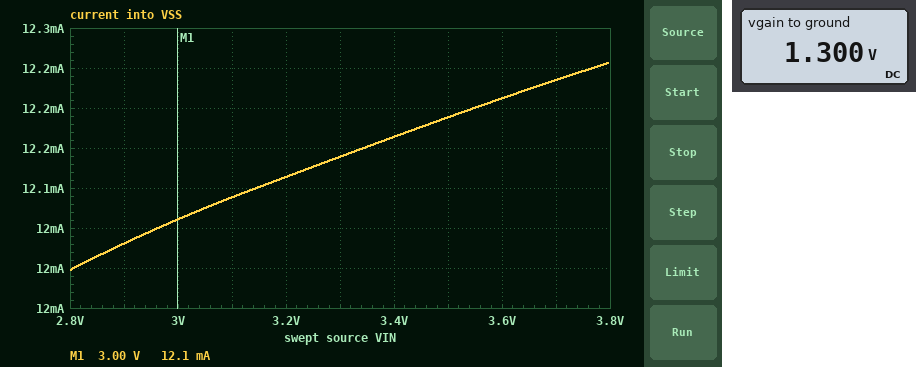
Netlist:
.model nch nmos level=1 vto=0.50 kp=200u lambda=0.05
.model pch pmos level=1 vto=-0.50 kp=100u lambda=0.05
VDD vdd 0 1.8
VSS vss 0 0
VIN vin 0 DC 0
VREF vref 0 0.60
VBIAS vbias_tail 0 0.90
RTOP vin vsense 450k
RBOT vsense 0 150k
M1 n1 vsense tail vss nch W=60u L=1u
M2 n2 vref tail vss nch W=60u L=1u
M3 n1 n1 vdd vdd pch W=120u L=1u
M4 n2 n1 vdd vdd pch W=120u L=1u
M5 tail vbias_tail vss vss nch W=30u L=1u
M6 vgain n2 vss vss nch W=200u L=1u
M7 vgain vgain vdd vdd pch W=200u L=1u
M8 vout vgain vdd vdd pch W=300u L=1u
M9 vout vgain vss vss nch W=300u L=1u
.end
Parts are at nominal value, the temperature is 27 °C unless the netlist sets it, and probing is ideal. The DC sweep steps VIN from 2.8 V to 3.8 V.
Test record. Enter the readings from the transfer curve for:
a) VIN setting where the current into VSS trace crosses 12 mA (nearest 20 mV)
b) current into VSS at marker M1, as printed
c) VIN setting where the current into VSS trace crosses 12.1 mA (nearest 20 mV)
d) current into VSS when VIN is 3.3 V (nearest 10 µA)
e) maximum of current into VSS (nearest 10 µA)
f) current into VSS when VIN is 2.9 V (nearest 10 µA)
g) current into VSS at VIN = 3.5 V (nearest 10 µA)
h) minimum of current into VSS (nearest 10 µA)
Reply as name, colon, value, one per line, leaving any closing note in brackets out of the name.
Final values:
VIN setting where the current into VSS trace crosses 12 mA: 2.96 V
current into VSS at marker M1, as printed: 12.1 mA
VIN setting where the current into VSS trace crosses 12.1 mA: 3.14 V
current into VSS when VIN is 3.3 V: 12.14 mA
maximum of current into VSS: 12.26 mA
current into VSS when VIN is 2.9 V: 12.03 mA
current into VSS at VIN = 3.5 V: 12.19 mA
minimum of current into VSS: 12.00 mA
